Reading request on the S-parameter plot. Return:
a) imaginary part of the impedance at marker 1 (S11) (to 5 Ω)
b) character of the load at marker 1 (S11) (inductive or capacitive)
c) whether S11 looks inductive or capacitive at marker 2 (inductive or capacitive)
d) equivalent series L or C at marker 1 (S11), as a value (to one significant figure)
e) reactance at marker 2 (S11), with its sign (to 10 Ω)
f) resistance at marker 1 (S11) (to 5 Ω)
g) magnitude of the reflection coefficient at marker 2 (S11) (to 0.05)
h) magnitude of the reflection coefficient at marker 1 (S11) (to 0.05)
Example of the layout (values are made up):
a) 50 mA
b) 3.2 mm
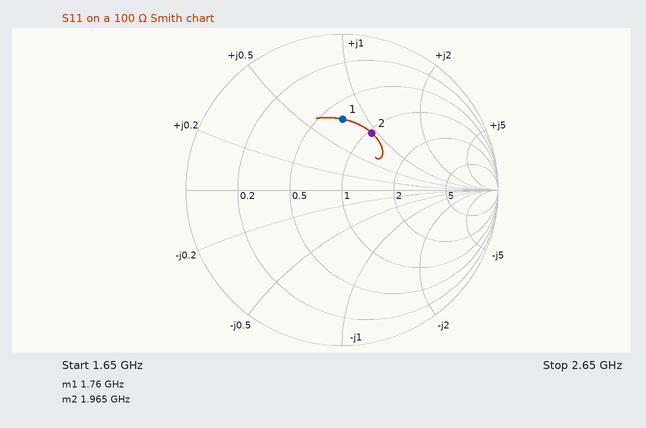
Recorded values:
a) +75 Ω
b) inductive
c) inductive
d) 7 nH
e) +90 Ω
f) 65 Ω
g) 0.40
h) 0.45
